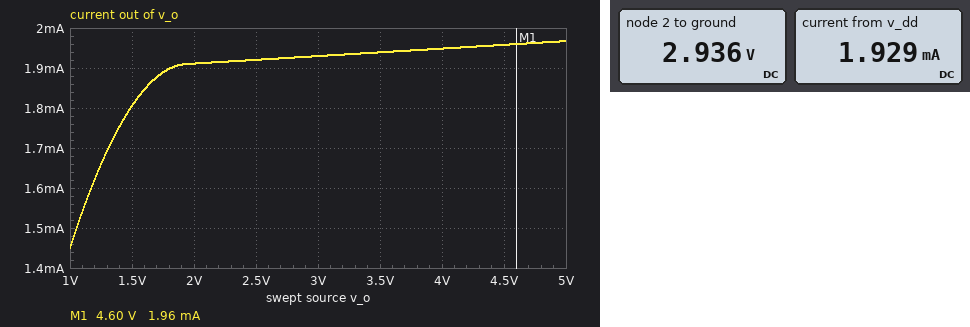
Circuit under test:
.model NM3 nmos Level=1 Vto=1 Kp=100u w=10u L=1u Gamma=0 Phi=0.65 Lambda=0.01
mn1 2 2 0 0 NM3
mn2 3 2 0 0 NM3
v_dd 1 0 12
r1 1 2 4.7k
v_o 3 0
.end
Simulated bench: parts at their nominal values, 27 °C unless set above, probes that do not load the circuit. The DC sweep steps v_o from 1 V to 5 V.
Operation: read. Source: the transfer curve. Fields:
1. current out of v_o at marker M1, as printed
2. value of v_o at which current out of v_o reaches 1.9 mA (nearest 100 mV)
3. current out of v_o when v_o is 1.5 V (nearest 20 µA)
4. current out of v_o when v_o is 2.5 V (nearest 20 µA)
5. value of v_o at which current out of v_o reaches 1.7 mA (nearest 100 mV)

1.96 mA
1.8 V
1.80 mA
1.92 mA
1.3 V
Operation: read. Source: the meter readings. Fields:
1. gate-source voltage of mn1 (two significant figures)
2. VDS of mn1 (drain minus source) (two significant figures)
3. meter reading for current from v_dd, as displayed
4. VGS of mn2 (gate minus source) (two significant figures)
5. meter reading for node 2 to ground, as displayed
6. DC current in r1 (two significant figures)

2.9 V
2.9 V
1.929 mA
2.9 V
2.936 V
1.9 mA
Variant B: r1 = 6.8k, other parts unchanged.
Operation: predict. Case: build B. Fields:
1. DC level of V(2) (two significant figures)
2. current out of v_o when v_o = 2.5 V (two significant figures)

2.6 V
1.4 mA
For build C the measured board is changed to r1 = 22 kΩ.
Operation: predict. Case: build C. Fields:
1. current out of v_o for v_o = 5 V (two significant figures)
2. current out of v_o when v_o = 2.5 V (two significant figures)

470 µA
460 µA
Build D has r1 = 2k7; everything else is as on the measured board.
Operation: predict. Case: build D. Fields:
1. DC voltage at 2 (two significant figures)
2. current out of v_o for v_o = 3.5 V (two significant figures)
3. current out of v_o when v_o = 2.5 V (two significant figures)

3.5 V
3.2 mA
3.1 mA
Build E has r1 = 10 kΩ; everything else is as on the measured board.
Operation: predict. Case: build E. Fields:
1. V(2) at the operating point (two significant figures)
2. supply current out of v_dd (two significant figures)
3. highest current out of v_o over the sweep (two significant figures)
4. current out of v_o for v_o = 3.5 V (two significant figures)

2.4 V
960 µA
990 µA
970 µA
